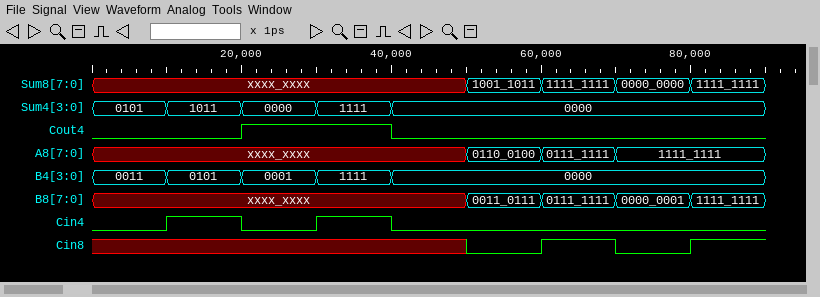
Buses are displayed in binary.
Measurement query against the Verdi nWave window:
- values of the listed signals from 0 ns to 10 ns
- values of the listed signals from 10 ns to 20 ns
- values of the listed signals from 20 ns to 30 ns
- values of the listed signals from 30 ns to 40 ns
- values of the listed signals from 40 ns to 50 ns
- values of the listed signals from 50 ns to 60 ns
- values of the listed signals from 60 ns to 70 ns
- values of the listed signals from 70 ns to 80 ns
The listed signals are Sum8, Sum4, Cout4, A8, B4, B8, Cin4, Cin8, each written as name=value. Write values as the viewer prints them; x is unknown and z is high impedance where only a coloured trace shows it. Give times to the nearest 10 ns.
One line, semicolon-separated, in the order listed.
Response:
Sum8=xxxx_xxxx, Sum4=0101, Cout4=0, A8=xxxx_xxxx, B4=0011, B8=xxxx_xxxx, Cin4=0, Cin8=x; Sum8=xxxx_xxxx, Sum4=1011, Cout4=0, A8=xxxx_xxxx, B4=0101, B8=xxxx_xxxx, Cin4=1, Cin8=x; Sum8=xxxx_xxxx, Sum4=0000, Cout4=1, A8=xxxx_xxxx, B4=0001, B8=xxxx_xxxx, Cin4=0, Cin8=x; Sum8=xxxx_xxxx, Sum4=1111, Cout4=1, A8=xxxx_xxxx, B4=1111, B8=xxxx_xxxx, Cin4=1, Cin8=x; Sum8=xxxx_xxxx, Sum4=0000, Cout4=0, A8=xxxx_xxxx, B4=0000, B8=xxxx_xxxx, Cin4=0, Cin8=x; Sum8=1001_1011, Sum4=0000, Cout4=0, A8=0110_0100, B4=0000, B8=0011_0111, Cin4=0, Cin8=0; Sum8=1111_1111, Sum4=0000, Cout4=0, A8=0111_1111, B4=0000, B8=0111_1111, Cin4=0, Cin8=1; Sum8=0000_0000, Sum4=0000, Cout4=0, A8=1111_1111, B4=0000, B8=0000_0001, Cin4=0, Cin8=0
